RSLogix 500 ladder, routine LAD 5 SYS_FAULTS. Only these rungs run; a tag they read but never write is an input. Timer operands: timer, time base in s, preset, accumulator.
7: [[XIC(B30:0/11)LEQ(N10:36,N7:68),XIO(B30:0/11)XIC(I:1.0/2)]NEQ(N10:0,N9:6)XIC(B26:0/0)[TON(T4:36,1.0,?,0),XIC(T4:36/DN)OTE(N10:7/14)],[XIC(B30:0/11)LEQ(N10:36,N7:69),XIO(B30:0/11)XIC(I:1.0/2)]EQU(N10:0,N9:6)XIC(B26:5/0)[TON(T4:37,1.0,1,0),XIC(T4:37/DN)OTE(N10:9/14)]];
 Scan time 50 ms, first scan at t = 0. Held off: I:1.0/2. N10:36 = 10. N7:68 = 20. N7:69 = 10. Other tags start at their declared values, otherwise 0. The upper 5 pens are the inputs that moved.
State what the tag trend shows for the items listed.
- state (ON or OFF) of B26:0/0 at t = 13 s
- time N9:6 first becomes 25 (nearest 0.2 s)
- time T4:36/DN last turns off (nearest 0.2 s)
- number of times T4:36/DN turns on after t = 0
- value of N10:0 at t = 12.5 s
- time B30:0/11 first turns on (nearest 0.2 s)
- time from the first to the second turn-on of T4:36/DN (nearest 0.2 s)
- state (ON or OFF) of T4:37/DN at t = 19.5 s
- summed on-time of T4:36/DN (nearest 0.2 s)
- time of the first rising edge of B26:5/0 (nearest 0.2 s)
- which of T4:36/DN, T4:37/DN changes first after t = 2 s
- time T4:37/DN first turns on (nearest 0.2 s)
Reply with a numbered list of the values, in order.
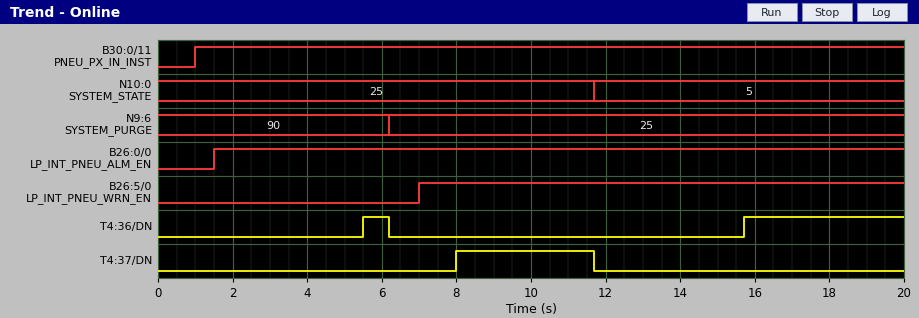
1. ON
2. 6.2 s
3. 6.2 s
4. 2
5. 5
6. 1.0 s
7. 10.2 s
8. OFF
9. 5.0 s
10. 7.0 s
11. T4:36/DN
12. 8.0 s
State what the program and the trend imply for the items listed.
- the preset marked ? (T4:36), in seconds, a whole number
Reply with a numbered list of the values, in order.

1. 4 s
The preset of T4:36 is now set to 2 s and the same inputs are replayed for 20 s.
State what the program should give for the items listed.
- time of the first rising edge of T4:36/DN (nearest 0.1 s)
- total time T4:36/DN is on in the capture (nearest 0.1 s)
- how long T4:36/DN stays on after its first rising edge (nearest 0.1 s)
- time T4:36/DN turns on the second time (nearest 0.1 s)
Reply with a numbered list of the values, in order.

1. 3.5 s
2. 9.0 s
3. 2.7 s
4. 13.7 s
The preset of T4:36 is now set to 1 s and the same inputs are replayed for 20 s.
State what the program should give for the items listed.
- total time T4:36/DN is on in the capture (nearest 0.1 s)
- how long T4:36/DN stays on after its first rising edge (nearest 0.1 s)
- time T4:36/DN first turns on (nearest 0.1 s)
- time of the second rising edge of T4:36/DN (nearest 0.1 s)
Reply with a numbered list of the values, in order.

1. 11.0 s
2. 3.7 s
3. 2.5 s
4. 12.7 s
